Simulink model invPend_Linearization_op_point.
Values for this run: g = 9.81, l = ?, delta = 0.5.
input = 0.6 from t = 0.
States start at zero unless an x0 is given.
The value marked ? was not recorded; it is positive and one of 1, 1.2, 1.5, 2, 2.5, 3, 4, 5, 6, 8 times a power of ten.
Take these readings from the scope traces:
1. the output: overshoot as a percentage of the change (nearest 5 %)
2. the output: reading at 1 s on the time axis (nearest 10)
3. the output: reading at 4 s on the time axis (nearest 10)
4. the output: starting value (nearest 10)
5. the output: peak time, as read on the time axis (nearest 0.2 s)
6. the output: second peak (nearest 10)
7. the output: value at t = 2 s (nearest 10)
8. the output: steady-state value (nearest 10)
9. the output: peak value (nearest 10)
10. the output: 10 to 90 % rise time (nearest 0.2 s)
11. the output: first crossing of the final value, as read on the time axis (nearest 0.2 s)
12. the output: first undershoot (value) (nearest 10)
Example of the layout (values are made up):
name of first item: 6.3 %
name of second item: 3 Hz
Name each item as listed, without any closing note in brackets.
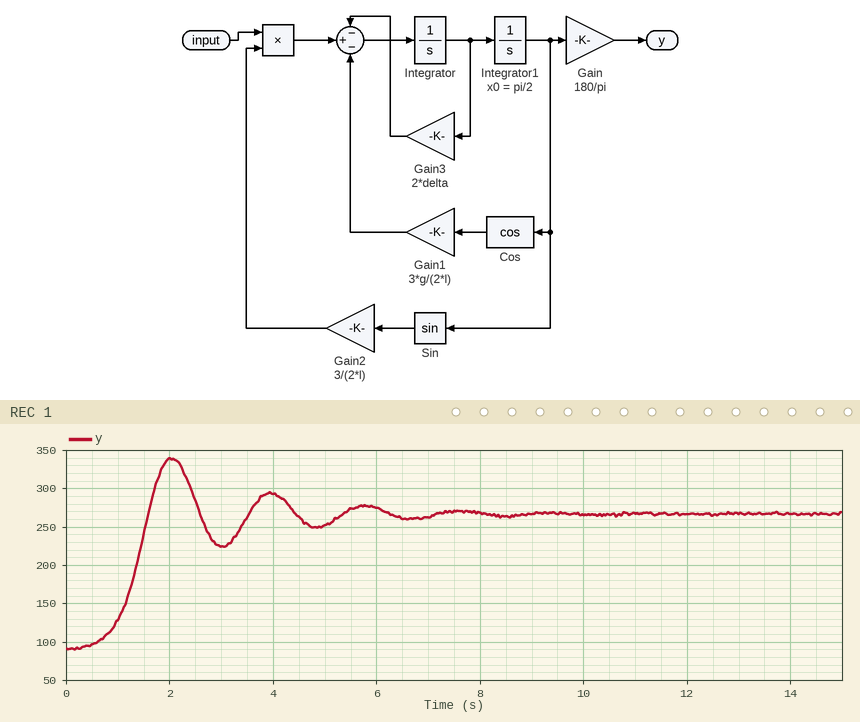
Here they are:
the output: overshoot as a percentage of the change: 40 %
the output: reading at 1 s on the time axis: 130
the output: reading at 4 s on the time axis: 290
the output: starting value: 90
the output: peak time, as read on the time axis: 2.0 s
the output: second peak: 290
the output: value at t = 2 s: 340
the output: steady-state value: 270
the output: peak value: 340
the output: 10 to 90 % rise time: 0.8 s
the output: first crossing of the final value, as read on the time axis: 1.6 s
the output: first undershoot (value): 220
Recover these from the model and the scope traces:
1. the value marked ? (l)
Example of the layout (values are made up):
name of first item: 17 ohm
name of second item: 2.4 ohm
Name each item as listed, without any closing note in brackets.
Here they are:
the value marked ?: 1.2
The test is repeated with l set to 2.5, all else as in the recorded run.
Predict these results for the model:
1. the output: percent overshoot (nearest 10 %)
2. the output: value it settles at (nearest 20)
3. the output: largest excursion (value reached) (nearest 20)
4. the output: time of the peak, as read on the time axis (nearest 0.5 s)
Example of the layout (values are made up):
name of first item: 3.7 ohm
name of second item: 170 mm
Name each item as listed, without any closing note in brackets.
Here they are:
the output: percent overshoot: 30 %
the output: value it settles at: 260
the output: largest excursion (value reached): 320
the output: time of the peak, as read on the time axis: 3.0 s
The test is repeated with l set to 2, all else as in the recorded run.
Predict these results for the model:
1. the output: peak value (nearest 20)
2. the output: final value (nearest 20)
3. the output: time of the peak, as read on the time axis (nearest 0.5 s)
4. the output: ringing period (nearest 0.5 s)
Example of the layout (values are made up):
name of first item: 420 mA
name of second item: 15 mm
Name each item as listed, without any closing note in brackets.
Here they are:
the output: peak value: 320
the output: final value: 260
the output: time of the peak, as read on the time axis: 2.5 s
the output: ringing period: 2.5 s
